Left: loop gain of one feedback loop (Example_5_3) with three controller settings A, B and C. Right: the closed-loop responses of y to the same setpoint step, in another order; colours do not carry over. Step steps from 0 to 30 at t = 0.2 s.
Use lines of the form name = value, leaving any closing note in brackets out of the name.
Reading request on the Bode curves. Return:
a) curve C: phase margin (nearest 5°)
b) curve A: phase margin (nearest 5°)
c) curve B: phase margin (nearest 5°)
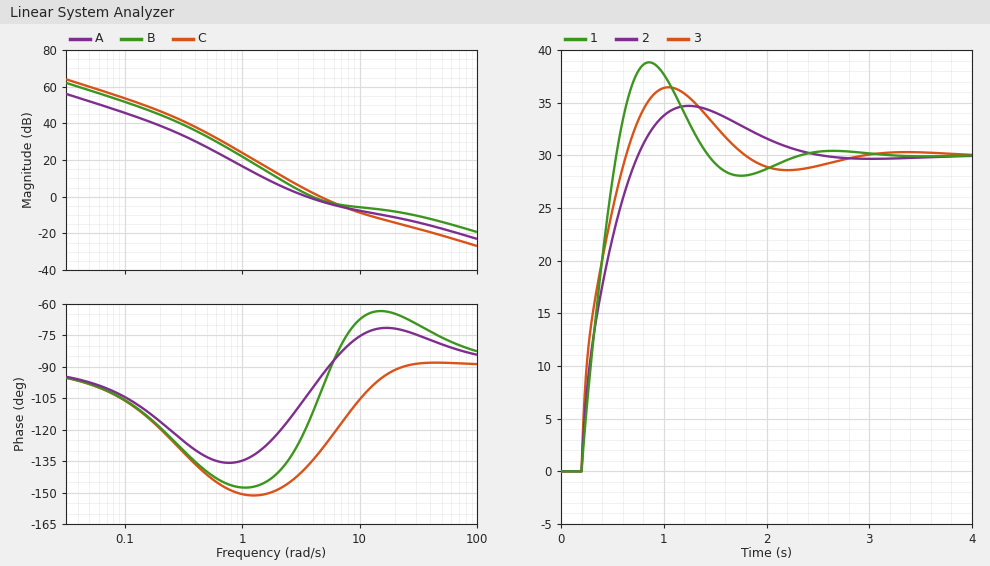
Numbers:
curve C: phase margin = 50°
curve A: phase margin = 75°
curve B: phase margin = 70°
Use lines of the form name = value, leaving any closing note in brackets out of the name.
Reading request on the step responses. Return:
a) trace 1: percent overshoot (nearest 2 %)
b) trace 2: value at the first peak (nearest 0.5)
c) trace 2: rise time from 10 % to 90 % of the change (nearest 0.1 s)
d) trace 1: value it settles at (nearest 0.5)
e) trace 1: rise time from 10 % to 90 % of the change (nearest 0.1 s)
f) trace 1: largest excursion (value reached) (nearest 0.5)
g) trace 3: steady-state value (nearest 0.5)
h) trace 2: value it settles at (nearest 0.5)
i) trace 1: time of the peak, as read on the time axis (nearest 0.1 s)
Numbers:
trace 1: percent overshoot = 30 %
trace 2: value at the first peak = 34.5
trace 2: rise time from 10 % to 90 % of the change = 0.4 s
trace 1: value it settles at = 30.0
trace 1: rise time from 10 % to 90 % of the change = 0.3 s
trace 1: largest excursion (value reached) = 39.0
trace 3: steady-state value = 30.0
trace 2: value it settles at = 30.0
trace 1: time of the peak, as read on the time axis = 0.9 s
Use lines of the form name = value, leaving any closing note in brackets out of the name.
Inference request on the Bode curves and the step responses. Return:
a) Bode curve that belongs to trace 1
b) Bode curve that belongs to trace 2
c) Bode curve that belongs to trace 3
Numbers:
Bode curve that belongs to trace 1 = C
Bode curve that belongs to trace 2 = A
Bode curve that belongs to trace 3 = B
